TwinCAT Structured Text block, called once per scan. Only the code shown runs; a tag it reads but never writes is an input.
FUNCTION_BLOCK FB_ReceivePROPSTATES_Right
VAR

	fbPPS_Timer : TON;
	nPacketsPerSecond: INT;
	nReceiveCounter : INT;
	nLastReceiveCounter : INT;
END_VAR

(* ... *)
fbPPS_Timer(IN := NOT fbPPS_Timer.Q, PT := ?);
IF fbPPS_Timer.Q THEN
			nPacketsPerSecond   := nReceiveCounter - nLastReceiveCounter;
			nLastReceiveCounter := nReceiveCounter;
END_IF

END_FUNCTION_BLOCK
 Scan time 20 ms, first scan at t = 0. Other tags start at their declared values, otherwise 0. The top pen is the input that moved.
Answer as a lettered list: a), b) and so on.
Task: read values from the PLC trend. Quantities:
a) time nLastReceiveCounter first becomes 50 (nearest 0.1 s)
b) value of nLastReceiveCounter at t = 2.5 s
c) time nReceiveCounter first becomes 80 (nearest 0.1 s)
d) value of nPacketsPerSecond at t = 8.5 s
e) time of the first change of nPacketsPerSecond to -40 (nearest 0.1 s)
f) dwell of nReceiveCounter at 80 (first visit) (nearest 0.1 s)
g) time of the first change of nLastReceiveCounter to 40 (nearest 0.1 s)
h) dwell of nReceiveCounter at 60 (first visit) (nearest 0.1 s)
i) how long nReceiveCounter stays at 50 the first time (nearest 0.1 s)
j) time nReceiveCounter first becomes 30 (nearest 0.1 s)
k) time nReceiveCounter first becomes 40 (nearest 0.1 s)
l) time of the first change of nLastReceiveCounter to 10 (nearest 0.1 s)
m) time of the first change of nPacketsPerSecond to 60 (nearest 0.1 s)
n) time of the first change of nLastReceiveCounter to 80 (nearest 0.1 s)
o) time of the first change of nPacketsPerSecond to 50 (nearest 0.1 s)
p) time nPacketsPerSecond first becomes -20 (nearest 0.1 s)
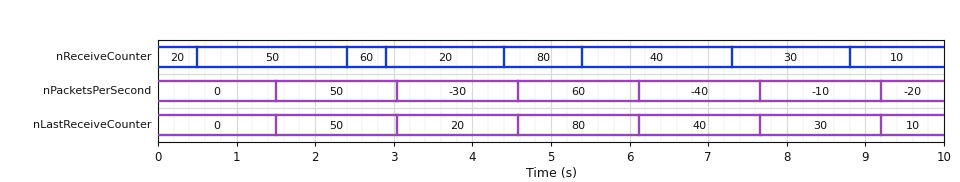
a) 1.5 s
b) 50
c) 4.4 s
d) -10
e) 6.1 s
f) 1.0 s
g) 6.1 s
h) 0.5 s
i) 1.9 s
j) 7.3 s
k) 5.4 s
l) 9.2 s
m) 4.6 s
n) 4.6 s
o) 1.5 s
p) 9.2 s
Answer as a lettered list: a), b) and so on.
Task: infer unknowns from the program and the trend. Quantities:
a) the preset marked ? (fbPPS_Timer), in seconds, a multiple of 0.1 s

a) 1.5 s
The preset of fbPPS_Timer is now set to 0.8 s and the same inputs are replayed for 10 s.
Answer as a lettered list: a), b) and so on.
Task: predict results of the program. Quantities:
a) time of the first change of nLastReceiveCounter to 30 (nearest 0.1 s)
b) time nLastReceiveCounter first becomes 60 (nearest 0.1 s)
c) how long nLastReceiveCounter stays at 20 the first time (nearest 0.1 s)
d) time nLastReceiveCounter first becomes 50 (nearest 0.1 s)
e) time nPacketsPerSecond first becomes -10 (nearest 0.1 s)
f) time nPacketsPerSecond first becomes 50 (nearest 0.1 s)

a) 7.5 s
b) 2.5 s
c) 1.7 s
d) 0.8 s
e) 7.5 s
f) 0.8 s
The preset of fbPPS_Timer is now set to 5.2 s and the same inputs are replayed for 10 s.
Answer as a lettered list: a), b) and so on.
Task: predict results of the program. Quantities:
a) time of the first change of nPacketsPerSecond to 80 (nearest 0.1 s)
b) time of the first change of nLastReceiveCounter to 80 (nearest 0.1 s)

a) 5.2 s
b) 5.2 s
